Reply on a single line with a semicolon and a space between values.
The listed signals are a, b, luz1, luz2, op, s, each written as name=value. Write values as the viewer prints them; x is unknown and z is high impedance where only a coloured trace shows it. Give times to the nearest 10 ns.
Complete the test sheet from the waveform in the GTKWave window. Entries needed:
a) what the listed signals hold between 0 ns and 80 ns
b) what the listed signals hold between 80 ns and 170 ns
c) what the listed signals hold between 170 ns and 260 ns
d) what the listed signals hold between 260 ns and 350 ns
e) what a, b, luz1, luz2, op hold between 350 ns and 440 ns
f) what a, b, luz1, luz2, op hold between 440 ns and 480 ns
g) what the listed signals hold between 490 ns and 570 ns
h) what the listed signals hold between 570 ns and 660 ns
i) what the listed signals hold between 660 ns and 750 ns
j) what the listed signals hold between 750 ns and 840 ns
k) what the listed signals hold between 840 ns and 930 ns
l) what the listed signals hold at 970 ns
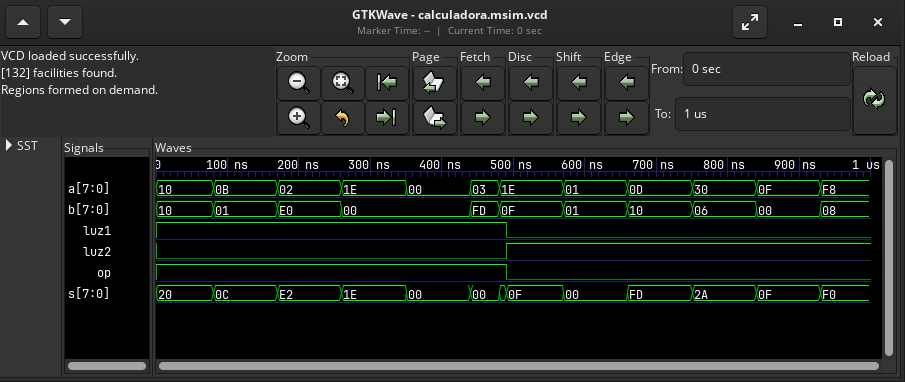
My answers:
a=10, b=10, luz1=1, luz2=0, op=1, s=20; a=0B, b=01, luz1=1, luz2=0, op=1, s=0C; a=02, b=E0, luz1=1, luz2=0, op=1, s=E2; a=1E, b=00, luz1=1, luz2=0, op=1, s=1E; a=00, b=00, luz1=1, luz2=0, op=1; a=03, b=FD, luz1=1, luz2=0, op=1; a=1E, b=0F, luz1=0, luz2=1, op=0, s=0F; a=01, b=01, luz1=0, luz2=1, op=0, s=00; a=0D, b=10, luz1=0, luz2=1, op=0, s=FD; a=30, b=06, luz1=0, luz2=1, op=0, s=2A; a=0F, b=00, luz1=0, luz2=1, op=0, s=0F; a=F8, b=08, luz1=0, luz2=1, op=0, s=F0
